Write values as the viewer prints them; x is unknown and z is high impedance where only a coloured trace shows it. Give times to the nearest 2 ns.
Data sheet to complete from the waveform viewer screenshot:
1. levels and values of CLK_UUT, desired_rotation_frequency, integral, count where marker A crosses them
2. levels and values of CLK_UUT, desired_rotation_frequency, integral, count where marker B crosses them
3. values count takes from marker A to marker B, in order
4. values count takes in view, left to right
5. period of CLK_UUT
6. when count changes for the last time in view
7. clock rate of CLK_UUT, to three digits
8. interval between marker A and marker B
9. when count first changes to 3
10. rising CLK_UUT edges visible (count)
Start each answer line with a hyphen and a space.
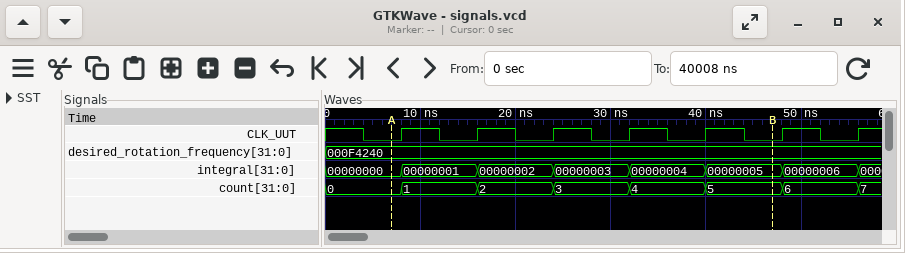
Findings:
- CLK_UUT=0, desired_rotation_frequency=000F4240, integral=00000000, count=0
- CLK_UUT=0, desired_rotation_frequency=000F4240, integral=00000005, count=5
- 0, 1, 2, 3, 4, 5
- 0, 1, 2, 3, 4, 5, 6, 7
- 8 ns
- 56 ns
- 125 MHz
- 40 ns
- 24 ns
- 7
